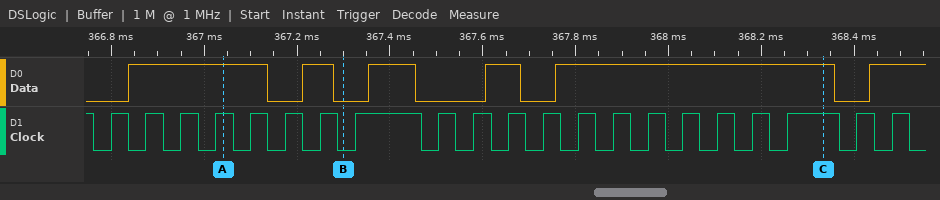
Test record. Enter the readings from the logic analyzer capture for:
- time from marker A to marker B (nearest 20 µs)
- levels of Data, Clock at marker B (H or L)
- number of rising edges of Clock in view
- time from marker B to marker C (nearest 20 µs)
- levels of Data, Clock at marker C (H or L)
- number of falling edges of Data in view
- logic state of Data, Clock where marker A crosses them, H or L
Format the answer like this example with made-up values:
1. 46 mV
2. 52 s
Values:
1. 260 µs
2. Data=L, Clock=L
3. 21
4. 1040 µs
5. Data=H, Clock=H
6. 5
7. Data=H, Clock=H
